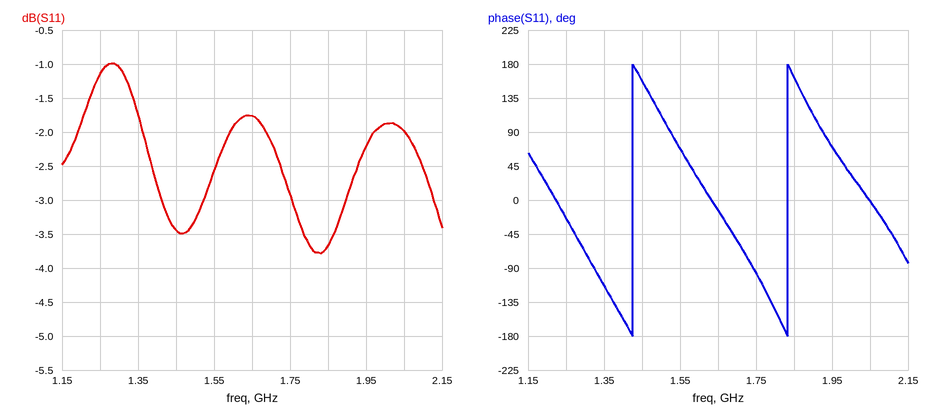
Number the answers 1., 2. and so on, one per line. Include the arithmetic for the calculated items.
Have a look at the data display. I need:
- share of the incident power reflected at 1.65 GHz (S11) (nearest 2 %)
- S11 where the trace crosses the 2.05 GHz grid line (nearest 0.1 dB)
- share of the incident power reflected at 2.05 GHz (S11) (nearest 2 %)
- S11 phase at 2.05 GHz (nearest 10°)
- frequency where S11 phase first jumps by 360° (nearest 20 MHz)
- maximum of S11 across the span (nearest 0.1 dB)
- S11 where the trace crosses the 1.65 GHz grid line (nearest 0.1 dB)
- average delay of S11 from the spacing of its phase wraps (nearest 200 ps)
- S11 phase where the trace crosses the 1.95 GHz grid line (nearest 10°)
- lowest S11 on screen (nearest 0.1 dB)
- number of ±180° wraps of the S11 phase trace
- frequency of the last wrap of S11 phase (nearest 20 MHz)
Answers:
1. 10^(-1.8/10) ≈ 66 %
2. -2.0 dB
3. 10^(-2/10) ≈ 63.1 %, so 64 % to the nearest 2 %
4. 0°
5. 1.42 GHz
6. -1.0 dB
7. -1.8 dB
8. 1 cycle / (1.84 GHz − 1.42 GHz) ≈ 2.4 ns
9. 70°
10. -3.8 dB
11. 2
12. 1.84 GHz
